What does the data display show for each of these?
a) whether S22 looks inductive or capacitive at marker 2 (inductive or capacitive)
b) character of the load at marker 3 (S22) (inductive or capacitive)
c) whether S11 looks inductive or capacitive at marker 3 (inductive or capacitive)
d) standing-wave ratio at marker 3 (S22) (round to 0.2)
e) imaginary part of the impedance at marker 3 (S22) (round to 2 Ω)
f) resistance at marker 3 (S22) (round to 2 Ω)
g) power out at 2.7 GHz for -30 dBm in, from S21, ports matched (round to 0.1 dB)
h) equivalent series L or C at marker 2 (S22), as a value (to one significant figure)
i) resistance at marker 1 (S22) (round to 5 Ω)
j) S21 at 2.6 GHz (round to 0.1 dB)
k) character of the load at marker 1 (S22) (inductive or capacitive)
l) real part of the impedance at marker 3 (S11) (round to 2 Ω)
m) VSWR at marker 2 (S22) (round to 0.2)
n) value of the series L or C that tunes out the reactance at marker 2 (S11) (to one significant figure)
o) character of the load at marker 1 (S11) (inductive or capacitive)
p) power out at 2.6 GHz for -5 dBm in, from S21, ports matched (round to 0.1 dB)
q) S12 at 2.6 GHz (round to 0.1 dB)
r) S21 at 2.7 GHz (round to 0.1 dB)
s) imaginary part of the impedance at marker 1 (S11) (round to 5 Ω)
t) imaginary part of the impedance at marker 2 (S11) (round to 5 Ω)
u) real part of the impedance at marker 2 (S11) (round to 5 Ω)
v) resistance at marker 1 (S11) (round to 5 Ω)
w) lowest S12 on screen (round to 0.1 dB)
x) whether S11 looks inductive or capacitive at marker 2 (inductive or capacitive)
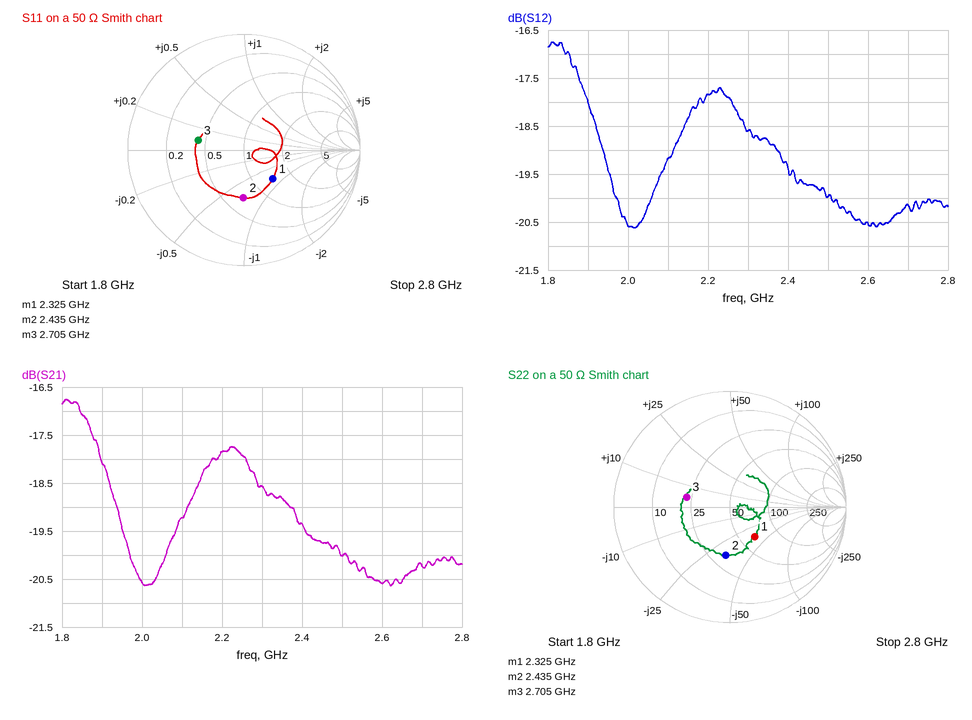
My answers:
capacitive
inductive
inductive
2.2
+4 Ω
22 Ω
-50.2 dBm
2 pF
65 Ω
-20.6 dB
capacitive
22 Ω
2.4
2 nH
capacitive
-25.6 dBm
-20.5 dB
-20.2 dB
-40 Ω
-35 Ω
35 Ω
70 Ω
-20.6 dB
capacitive
